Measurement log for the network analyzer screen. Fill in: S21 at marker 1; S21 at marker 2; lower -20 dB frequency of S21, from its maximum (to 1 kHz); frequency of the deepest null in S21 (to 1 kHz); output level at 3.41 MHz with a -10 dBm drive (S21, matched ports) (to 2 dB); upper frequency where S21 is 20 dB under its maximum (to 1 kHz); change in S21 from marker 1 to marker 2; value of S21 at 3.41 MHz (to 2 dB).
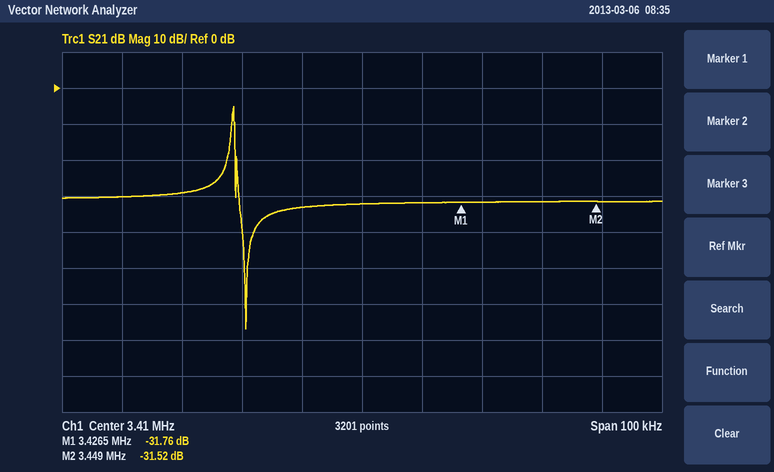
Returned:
-31.76 dB
-31.52 dB
3.386 MHz
3.391 MHz
-42 dBm
3.389 MHz
0.24 dB
-32 dB
